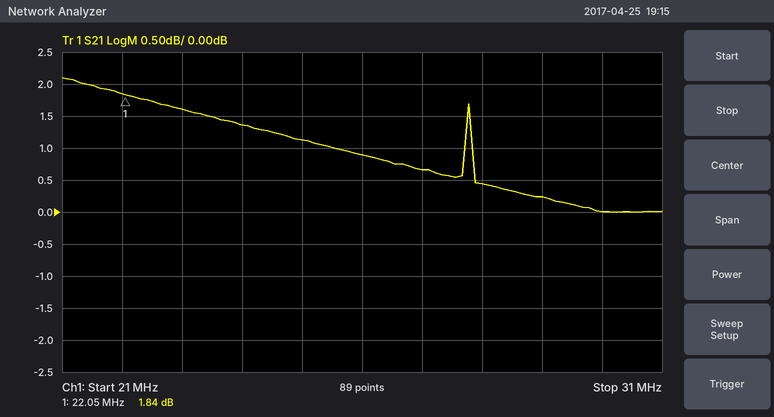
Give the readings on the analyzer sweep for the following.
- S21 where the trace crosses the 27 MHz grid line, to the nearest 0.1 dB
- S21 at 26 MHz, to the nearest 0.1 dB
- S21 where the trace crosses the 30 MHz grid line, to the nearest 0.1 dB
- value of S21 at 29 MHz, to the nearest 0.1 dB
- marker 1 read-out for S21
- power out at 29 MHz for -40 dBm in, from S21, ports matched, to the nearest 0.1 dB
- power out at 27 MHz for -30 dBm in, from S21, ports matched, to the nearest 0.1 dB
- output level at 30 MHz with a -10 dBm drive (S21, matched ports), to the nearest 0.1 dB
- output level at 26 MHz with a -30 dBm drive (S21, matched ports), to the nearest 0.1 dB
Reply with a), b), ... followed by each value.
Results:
a) 0.7 dB
b) 0.9 dB
c) 0.0 dB
d) 0.2 dB
e) 1.84 dB
f) -39.8 dBm
g) -29.3 dBm
h) -10.0 dBm
i) -29.1 dBm
